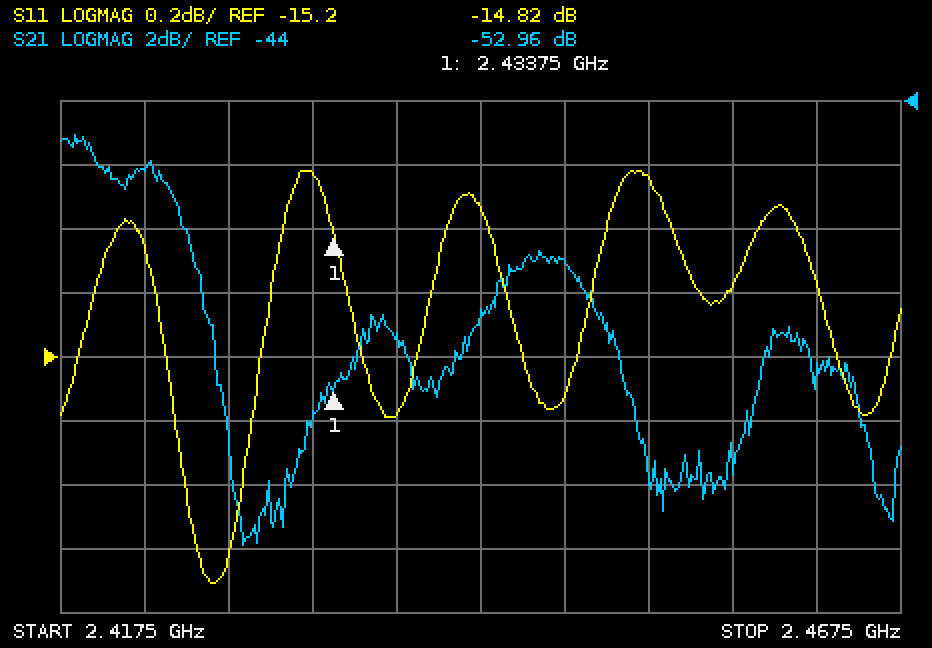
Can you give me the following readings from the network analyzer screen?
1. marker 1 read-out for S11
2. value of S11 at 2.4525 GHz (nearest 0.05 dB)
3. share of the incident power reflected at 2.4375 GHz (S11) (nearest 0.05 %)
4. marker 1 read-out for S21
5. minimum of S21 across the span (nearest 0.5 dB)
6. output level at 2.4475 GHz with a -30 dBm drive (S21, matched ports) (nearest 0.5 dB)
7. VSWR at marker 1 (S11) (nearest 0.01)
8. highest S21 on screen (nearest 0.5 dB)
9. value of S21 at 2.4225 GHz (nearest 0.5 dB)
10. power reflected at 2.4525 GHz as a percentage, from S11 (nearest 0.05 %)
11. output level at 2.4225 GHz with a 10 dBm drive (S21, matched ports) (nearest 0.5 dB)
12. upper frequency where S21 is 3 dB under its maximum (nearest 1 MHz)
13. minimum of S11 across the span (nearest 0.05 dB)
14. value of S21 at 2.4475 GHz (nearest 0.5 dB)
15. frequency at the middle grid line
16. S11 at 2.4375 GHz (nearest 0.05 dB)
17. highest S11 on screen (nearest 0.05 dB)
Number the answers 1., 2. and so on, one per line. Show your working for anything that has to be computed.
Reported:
1. -14.82 dB
2. -14.65 dB
3. 10^(-15.4/10) ≈ 2.88 %, so 2.90 % to the nearest 0.05 %
4. -52.96 dB
5. -58.0 dB
6. -30 dBm + (-49.0 dB) = -79.0 dBm
7. (1 + 0.1816)/(1 − 0.1816) ≈ 1.44
8. -45.0 dB
9. -46.0 dB
10. 10^(-14.65/10) ≈ 3.43 %, so 3.45 % to the nearest 0.05 %
11. 10 dBm + (-46.0 dB) = -36.0 dBm
12. 2.425 GHz
13. -15.90 dB
14. -49.0 dB
15. 2.4425 GHz
16. -15.40 dB
17. -14.60 dB
